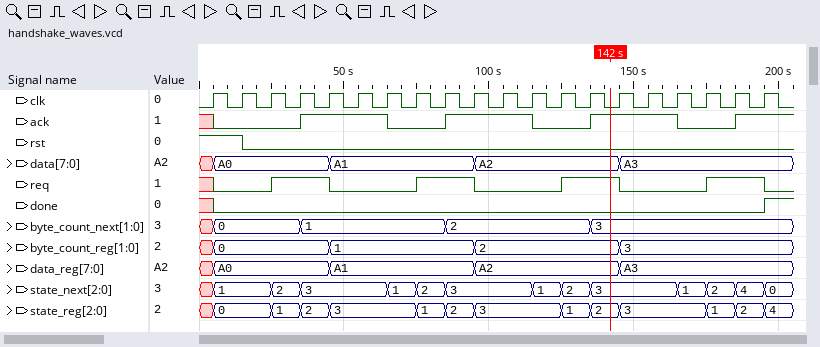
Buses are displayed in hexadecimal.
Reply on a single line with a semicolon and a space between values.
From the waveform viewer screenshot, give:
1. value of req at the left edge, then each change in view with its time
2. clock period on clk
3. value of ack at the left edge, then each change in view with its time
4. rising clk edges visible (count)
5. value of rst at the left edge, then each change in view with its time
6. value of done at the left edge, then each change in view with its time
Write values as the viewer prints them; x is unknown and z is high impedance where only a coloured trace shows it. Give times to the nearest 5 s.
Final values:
x, 0 at 5 s, 1 at 25 s, 0 at 45 s, 1 at 75 s, 0 at 95 s, 1 at 125 s, 0 at 145 s, 1 at 175 s, 0 at 195 s; 10 s; x, 0 at 5 s, 1 at 35 s, 0 at 65 s, 1 at 85 s, 0 at 115 s, 1 at 135 s, 0 at 165 s, 1 at 185 s; 20; 1, 0 at 15 s; x, 0 at 5 s, 1 at 195 s
